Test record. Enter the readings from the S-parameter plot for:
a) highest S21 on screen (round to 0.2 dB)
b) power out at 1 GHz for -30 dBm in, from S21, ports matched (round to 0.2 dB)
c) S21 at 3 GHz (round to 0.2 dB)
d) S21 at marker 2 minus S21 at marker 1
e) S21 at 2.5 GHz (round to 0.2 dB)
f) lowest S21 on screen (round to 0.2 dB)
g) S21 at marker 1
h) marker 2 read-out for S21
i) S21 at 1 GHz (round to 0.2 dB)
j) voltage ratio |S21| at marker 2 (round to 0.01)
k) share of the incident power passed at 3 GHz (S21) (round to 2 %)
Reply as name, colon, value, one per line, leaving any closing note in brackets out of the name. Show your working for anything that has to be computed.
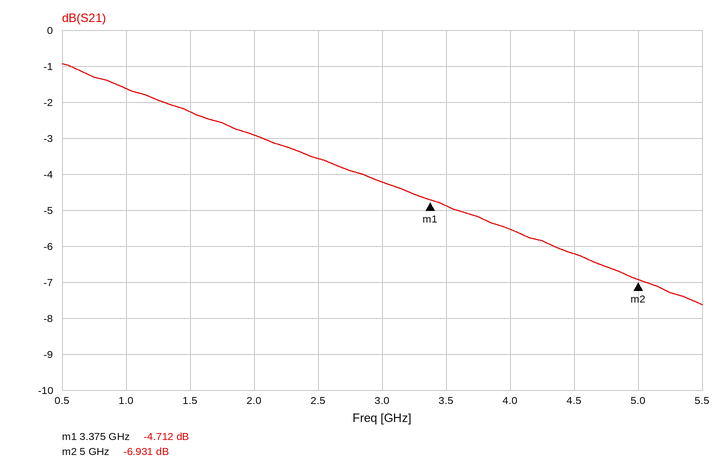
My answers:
highest S21 on screen: -1.0 dB
power out at 1 GHz for -30 dBm in, from S21, ports matched: -30 dBm + (-1.6 dB) = -31.6 dBm
S21 at 3 GHz: -4.2 dB
S21 at marker 2 minus S21 at marker 1: -6.931 − (-4.712) = -2.219 dB
S21 at 2.5 GHz: -3.6 dB
lowest S21 on screen: -7.6 dB
S21 at marker 1: -4.712 dB
marker 2 read-out for S21: -6.931 dB
S21 at 1 GHz: -1.6 dB
voltage ratio |S21| at marker 2: 10^(-6.931/20) ≈ 0.45
share of the incident power passed at 3 GHz (S21): 10^(-4.2/10) ≈ 38 %
